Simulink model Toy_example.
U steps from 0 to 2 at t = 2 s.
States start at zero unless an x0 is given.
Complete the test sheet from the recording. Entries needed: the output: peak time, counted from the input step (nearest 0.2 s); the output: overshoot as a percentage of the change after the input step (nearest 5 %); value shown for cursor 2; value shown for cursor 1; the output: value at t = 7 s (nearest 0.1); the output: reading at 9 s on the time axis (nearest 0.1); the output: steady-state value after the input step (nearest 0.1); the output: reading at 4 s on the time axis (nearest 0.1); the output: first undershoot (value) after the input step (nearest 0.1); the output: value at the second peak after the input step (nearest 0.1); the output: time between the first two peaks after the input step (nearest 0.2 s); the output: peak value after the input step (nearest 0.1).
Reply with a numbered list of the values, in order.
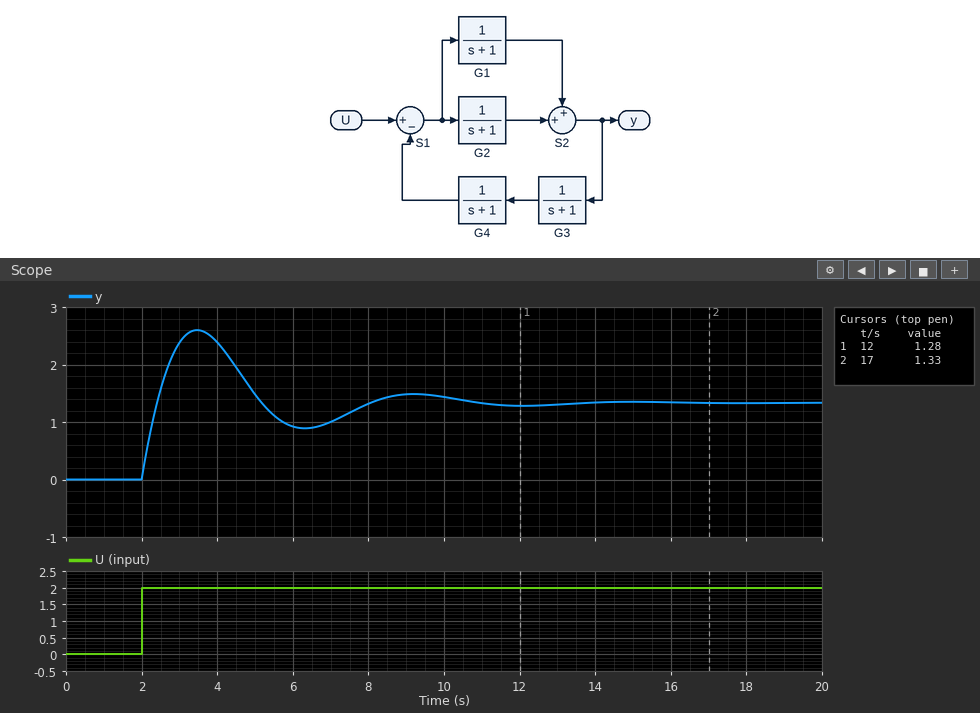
1. 1.4 s
2. 95 %
3. 1.33
4. 1.28
5. 1.0
6. 1.5
7. 1.3
8. 2.4
9. 0.9
10. 1.5
11. 5.8 s
12. 2.6
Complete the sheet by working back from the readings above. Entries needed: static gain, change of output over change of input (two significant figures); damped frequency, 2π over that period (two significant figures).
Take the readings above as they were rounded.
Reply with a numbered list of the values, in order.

1. 0.65
2. 1.1 rad/s
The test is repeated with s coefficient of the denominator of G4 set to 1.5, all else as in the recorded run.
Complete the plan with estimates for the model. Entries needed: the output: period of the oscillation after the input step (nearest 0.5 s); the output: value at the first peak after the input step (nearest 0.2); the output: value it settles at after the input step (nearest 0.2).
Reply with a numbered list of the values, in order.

1. 6.5 s
2. 2.8
3. 1.4
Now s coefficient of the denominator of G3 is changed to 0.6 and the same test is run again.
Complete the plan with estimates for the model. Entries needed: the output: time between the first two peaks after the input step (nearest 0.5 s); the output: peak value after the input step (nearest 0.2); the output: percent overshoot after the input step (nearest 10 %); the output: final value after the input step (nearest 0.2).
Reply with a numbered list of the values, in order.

1. 5.0 s
2. 2.4
3. 80 %
4. 1.4
